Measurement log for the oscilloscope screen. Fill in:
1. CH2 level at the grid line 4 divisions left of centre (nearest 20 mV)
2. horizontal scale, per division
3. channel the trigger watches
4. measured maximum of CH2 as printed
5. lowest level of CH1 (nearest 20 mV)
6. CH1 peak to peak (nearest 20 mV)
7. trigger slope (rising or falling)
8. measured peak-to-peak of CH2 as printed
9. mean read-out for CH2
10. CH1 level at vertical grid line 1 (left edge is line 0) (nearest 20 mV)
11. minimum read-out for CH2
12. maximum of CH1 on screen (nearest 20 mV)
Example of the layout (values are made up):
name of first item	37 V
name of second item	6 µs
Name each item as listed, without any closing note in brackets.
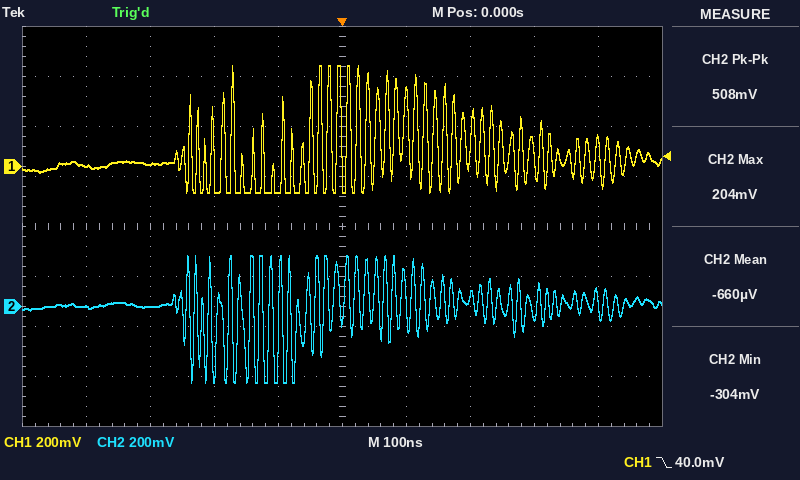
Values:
CH2 level at the grid line 4 divisions left of centre	0 mV
horizontal scale, per division	100 ns
channel the trigger watches	CH1
measured maximum of CH2 as printed	204 mV
lowest level of CH1	-100 mV
CH1 peak to peak	500 mV
trigger slope	falling
measured peak-to-peak of CH2 as printed	508 mV
mean read-out for CH2	-660 µV
CH1 level at vertical grid line 1 (left edge is line 0)	0 mV
minimum read-out for CH2	-304 mV
maximum of CH1 on screen	400 mV
